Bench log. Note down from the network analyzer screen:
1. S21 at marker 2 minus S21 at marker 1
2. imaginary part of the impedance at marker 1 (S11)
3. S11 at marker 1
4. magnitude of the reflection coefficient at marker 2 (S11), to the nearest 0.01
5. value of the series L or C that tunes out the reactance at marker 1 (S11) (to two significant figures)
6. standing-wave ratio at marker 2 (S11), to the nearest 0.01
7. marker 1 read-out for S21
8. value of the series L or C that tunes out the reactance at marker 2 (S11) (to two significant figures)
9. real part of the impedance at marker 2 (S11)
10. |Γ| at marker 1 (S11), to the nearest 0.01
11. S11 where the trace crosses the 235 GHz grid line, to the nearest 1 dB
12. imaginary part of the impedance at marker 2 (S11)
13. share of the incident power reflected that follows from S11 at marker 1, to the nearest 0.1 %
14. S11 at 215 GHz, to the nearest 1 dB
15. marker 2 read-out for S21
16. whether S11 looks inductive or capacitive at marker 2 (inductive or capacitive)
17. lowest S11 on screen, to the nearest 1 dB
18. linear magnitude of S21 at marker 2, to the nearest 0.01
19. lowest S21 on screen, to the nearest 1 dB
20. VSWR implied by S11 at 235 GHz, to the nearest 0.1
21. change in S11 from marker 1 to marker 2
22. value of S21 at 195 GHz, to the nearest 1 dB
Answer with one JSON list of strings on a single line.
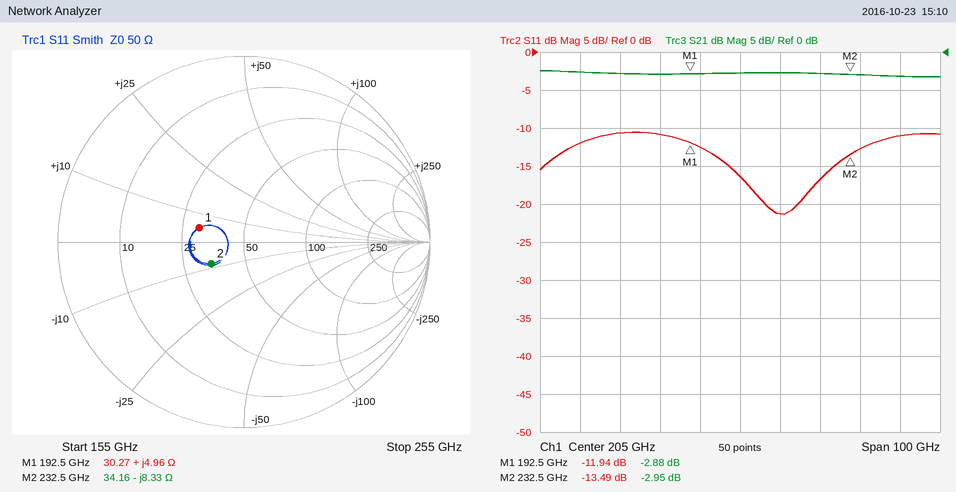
["-0.07 dB", "+4.96 Ω", "-11.94 dB", "0.21", "170 fF", "1.54", "-2.88 dB", "5.7 pH", "34.16 Ω", "0.25", "-13 dB", "-8.33 Ω", "6.4 %", "-21 dB", "-2.95 dB", "capacitive", "-21 dB", "0.71", "-3 dB", "1.6", "-1.55 dB", "-3 dB"]
